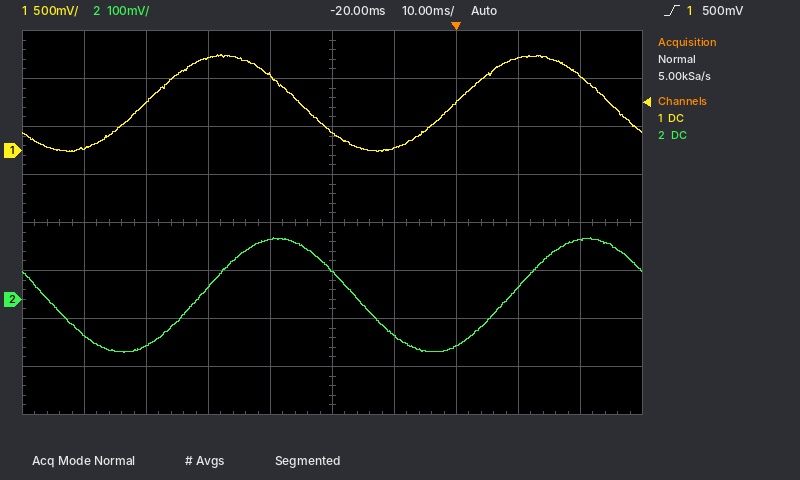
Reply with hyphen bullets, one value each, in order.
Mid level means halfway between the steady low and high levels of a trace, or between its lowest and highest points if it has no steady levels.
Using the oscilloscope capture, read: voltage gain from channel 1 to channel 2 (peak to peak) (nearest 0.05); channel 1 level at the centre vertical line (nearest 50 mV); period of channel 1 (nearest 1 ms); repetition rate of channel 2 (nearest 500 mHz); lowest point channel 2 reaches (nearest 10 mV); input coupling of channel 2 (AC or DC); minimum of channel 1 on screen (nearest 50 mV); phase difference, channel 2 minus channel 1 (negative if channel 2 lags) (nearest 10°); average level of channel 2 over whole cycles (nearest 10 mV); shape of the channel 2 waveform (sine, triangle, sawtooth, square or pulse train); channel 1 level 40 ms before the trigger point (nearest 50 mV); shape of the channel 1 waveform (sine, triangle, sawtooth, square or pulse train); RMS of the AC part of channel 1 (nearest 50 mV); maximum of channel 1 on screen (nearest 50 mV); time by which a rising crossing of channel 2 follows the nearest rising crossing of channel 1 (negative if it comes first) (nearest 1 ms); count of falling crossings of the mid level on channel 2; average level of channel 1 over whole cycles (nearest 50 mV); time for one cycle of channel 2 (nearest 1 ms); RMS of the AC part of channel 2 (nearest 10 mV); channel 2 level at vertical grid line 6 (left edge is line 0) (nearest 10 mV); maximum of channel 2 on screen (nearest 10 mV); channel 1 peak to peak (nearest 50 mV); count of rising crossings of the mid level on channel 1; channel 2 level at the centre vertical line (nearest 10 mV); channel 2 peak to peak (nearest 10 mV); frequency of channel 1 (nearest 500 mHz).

- 0.25
- 200 mV
- 50 ms
- 20.0 Hz
- -110 mV
- DC
- 0 mV
- -60°
- 10 mV
- sine
- 950 mV
- sine
- 350 mV
- 1.00 V
- +9 ms
- 2
- 500 mV
- 50 ms
- 80 mV
- -80 mV
- 130 mV
- 1.00 V
- 2
- 60 mV
- 240 mV
- 20.0 Hz
